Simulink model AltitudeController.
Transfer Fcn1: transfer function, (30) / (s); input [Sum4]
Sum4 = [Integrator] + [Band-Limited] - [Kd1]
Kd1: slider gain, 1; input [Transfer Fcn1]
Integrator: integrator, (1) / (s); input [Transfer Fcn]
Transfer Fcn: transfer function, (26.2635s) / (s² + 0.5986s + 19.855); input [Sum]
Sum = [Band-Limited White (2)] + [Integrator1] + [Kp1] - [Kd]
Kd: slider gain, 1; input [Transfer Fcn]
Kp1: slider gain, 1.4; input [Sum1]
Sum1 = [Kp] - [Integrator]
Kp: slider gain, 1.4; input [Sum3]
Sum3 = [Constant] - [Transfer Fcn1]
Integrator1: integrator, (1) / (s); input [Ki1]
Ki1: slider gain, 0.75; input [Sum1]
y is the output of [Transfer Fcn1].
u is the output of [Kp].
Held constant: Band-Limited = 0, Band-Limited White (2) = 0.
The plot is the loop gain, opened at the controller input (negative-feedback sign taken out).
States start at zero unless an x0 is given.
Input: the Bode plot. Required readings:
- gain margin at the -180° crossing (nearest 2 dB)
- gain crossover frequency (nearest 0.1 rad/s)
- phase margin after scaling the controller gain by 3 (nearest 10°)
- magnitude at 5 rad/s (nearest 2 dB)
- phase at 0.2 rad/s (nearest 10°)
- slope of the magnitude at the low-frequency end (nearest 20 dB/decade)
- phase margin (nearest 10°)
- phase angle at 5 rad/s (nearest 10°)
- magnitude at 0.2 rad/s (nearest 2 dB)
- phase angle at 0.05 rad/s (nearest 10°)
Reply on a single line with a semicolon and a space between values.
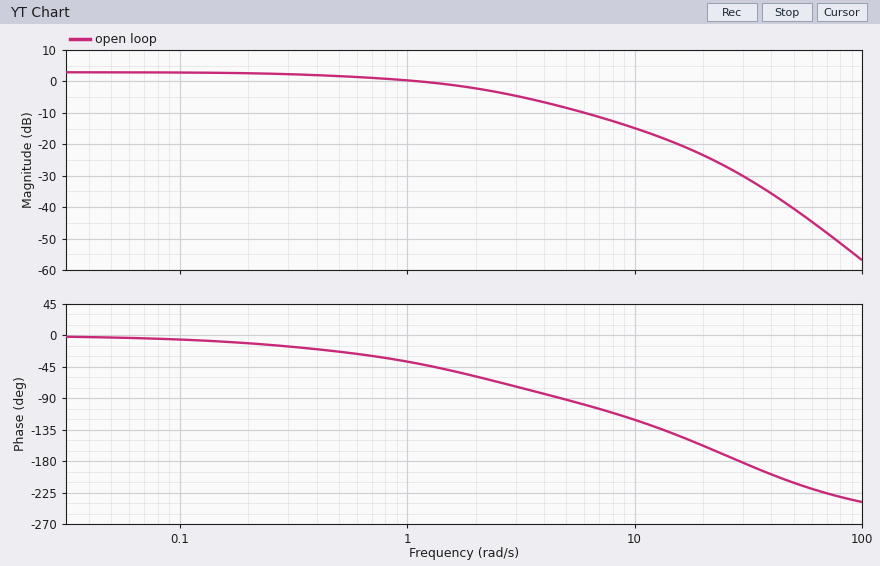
30 dB; 1.1 rad/s; 80°; -8 dB; -10°; 0 dB/decade; 140°; -90°; 2 dB; 0°
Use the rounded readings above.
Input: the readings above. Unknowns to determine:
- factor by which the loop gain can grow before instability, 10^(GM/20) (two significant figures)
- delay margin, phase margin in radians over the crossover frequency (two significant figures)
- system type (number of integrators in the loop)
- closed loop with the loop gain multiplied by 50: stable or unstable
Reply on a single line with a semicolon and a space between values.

32; 2.2 s; 0; unstable
